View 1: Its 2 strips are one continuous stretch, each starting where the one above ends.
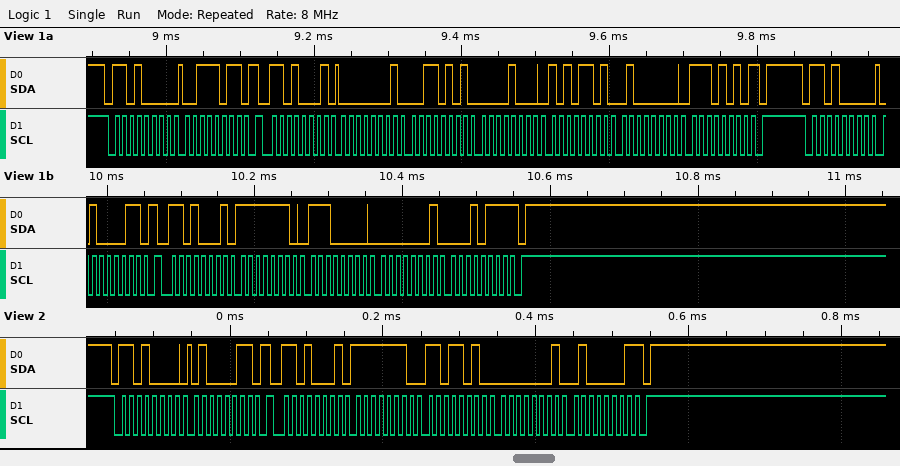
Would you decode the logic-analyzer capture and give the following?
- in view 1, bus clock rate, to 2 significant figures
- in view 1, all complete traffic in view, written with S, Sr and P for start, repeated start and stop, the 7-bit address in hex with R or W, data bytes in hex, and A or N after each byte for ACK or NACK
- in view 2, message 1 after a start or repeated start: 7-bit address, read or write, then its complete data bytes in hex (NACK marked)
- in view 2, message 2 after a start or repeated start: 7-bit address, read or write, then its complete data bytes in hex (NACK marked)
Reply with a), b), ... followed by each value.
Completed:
a) 100 kHz
b) S 68W A 3B A Sr 68R A 01 A 35 A 08 A AD A 40 A EA N P S 68W A 43 A Sr 68R A FE A E0 A 01 A 17 N P
c) 0x68 write: 43
d) 0x68 read: FE DA 01 41 NACK
